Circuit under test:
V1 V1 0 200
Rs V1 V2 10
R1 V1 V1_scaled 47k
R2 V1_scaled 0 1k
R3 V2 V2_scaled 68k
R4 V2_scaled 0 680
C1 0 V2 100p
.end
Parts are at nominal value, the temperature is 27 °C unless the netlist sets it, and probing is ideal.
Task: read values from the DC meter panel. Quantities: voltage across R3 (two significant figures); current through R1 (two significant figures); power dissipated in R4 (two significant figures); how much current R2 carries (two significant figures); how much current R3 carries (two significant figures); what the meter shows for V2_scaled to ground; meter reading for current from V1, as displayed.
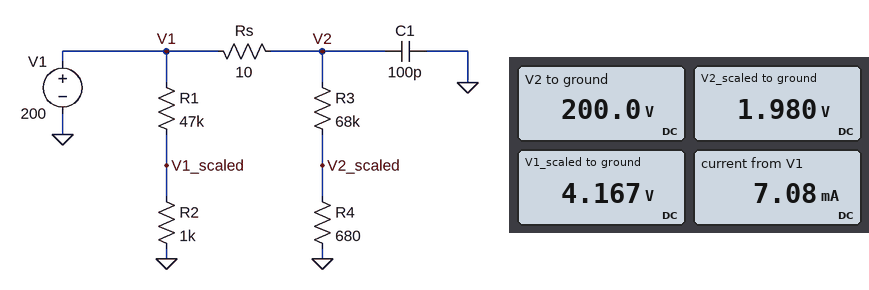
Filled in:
200 V
4.2 mA
5.8 mW
4.2 mA
2.9 mA
1.980 V
7.08 mA
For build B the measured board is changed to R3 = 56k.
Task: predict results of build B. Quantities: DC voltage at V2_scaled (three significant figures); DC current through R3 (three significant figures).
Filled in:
2.40 V
3.53 mA
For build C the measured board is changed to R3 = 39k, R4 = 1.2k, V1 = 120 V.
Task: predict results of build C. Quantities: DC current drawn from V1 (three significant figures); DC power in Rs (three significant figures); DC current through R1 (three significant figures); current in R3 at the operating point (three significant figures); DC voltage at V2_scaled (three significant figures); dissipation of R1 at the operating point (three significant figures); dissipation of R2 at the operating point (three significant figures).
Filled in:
5.48 mA
89.1 µW
2.50 mA
2.98 mA
3.58 V
294 mW
6.25 mW
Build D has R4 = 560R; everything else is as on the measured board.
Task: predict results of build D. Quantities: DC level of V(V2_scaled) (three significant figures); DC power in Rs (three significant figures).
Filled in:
1.63 V
85.1 µW
